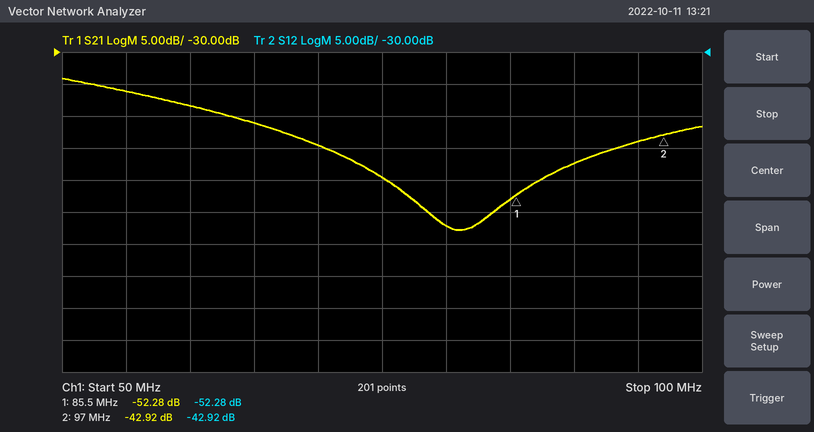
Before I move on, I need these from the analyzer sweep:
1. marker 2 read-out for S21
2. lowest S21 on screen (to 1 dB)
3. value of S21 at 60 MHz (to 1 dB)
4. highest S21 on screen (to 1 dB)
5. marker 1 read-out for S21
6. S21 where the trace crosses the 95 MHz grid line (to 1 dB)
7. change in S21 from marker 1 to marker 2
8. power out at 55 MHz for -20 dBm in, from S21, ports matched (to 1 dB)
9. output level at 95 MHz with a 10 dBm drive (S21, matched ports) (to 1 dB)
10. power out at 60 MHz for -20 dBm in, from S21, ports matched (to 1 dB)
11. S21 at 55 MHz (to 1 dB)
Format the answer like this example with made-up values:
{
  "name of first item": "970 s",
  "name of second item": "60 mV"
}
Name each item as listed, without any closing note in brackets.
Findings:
{
  "marker 2 read-out for S21": "-42.92 dB",
  "lowest S21 on screen": "-58 dB",
  "value of S21 at 60 MHz": "-38 dB",
  "highest S21 on screen": "-34 dB",
  "marker 1 read-out for S21": "-52.28 dB",
  "S21 where the trace crosses the 95 MHz grid line": "-44 dB",
  "change in S21 from marker 1 to marker 2": "9.36 dB",
  "power out at 55 MHz for -20 dBm in, from S21, ports matched": "-56 dBm",
  "output level at 95 MHz with a 10 dBm drive (S21, matched ports)": "-34 dBm",
  "power out at 60 MHz for -20 dBm in, from S21, ports matched": "-58 dBm",
  "S21 at 55 MHz": "-36 dB"
}
